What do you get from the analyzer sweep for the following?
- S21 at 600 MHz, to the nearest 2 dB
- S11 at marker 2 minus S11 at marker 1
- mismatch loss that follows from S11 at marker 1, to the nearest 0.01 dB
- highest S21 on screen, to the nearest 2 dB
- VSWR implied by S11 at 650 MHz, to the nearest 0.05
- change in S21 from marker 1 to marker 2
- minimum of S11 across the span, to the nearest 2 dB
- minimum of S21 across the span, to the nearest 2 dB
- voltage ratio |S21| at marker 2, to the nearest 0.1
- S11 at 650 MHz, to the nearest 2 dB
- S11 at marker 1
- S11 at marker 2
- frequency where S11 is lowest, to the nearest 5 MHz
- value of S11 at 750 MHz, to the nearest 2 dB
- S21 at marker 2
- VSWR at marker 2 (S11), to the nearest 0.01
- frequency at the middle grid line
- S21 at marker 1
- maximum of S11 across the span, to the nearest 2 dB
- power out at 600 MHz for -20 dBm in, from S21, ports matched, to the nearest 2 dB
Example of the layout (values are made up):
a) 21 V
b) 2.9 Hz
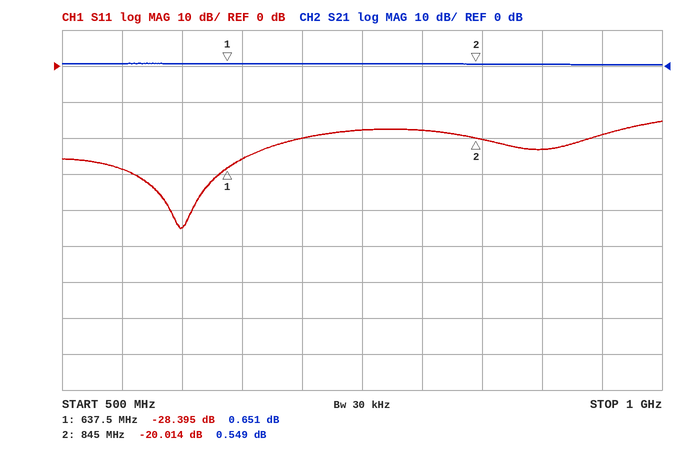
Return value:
a) 0 dB
b) 8.381 dB
c) 0.01 dB
d) 0 dB
e) 1.10
f) -0.102 dB
g) -46 dB
h) 0 dB
i) 1.1
j) -26 dB
k) -28.395 dB
l) -20.014 dB
m) 600 MHz
n) -18 dB
o) 0.549 dB
p) 1.22
q) 750 MHz
r) 0.651 dB
s) -16 dB
t) -20 dBm
